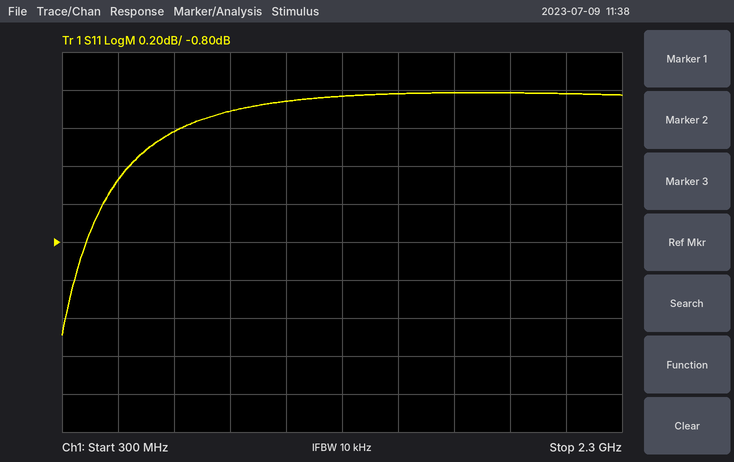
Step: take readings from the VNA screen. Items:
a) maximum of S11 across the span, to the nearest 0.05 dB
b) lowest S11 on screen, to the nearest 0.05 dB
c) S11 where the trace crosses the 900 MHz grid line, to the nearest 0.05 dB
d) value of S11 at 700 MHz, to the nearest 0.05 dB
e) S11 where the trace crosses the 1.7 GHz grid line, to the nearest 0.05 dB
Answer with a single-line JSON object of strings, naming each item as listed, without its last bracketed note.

{"maximum of S11 across the span, to the nearest 0.05 dB": "0.00 dB", "lowest S11 on screen, to the nearest 0.05 dB": "-1.30 dB", "S11 where the trace crosses the 900 MHz grid line, to the nearest 0.05 dB": "-0.10 dB", "value of S11 at 700 MHz, to the nearest 0.05 dB": "-0.20 dB", "S11 where the trace crosses the 1.7 GHz grid line, to the nearest 0.05 dB": "0.00 dB"}
